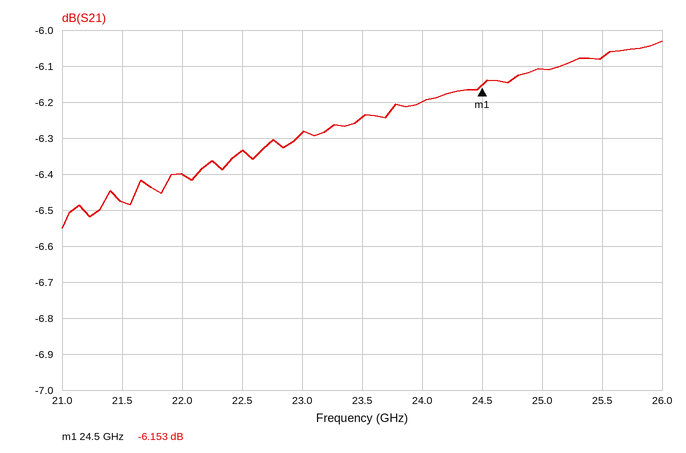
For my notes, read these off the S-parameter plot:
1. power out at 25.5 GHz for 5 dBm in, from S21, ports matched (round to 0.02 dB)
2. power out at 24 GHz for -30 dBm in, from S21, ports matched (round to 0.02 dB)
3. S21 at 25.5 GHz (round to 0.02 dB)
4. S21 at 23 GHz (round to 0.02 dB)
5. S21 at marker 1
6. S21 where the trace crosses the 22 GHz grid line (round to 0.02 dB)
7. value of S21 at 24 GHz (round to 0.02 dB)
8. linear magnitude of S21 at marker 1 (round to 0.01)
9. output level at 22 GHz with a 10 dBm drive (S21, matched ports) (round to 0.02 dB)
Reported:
-1.08 dBm
-36.20 dBm
-6.08 dB
-6.28 dB
-6.153 dB
-6.40 dB
-6.20 dB
0.49
3.60 dBm
